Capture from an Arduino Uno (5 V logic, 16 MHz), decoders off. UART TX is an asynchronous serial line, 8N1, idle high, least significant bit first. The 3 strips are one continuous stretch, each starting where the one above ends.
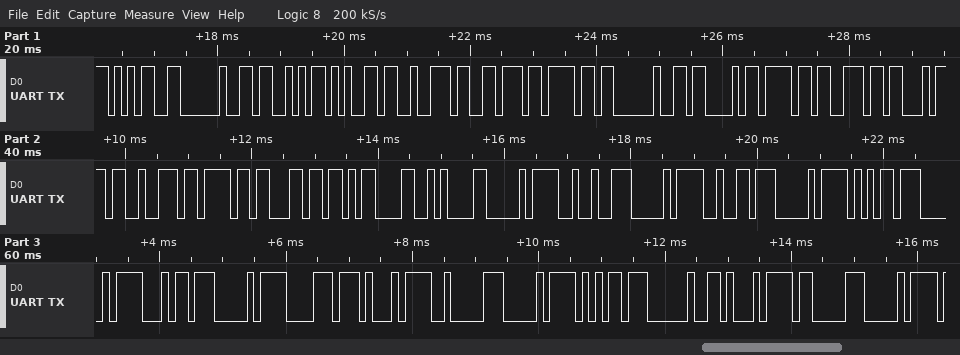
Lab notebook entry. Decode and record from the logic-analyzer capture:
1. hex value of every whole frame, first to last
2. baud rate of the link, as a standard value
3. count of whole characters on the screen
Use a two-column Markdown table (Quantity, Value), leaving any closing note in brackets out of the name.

| Quantity | Value |
|---|---|
| hex value of every whole frame, first to last | 35 20 53 65 72 76 6F 20 43 6F 6E 74 72 6F 6C 0D 0A D0 92 D0 B2 D0 B5 D0 B4 D0 B8 D1 82 D0 B5 20 D1 83 D0 |
| baud rate of the link, as a standard value | 9600 baud |
| count of whole characters on the screen | 35 |
